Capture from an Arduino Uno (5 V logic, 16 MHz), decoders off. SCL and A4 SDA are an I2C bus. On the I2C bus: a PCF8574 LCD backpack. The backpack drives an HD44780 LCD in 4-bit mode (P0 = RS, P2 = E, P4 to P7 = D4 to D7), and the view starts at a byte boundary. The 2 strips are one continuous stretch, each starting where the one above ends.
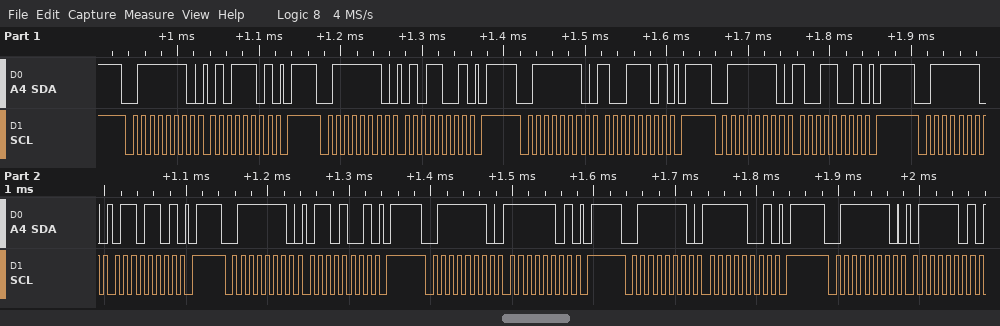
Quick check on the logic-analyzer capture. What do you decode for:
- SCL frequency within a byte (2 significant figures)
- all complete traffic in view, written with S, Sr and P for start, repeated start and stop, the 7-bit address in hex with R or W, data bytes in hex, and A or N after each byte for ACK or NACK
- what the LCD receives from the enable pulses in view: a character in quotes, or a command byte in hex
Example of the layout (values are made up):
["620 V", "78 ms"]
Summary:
["100 kHz", "S 3FW A 5D A P S 3FW A 59 A P S 3FW A 9D A P S 3FW A 99 A P S 3FW A 6D A P S 3FW A 69 A P S 3FW A FD A P S 3FW A F9 A P S 3FW A 7D A", "'Y' 'o'"]
